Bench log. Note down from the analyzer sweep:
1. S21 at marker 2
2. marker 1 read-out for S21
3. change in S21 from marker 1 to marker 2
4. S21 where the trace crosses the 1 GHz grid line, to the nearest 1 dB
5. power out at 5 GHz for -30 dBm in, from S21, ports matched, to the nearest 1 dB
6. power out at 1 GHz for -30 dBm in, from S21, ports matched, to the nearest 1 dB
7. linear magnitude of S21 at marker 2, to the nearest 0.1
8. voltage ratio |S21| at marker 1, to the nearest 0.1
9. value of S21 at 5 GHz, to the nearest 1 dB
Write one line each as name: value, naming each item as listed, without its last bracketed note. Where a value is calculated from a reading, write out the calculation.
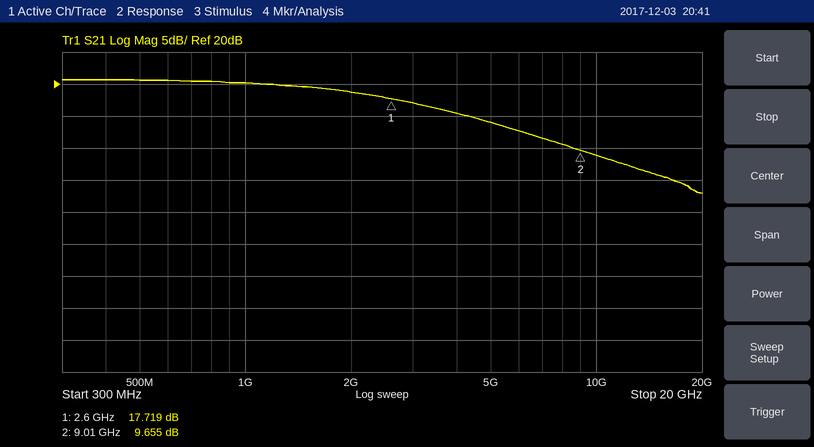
S21 at marker 2: 9.655 dB
marker 1 read-out for S21: 17.719 dB
change in S21 from marker 1 to marker 2: 9.655 − (17.719) = -8.064 dB
S21 where the trace crosses the 1 GHz grid line, to the nearest 1 dB: 20 dB
power out at 5 GHz for -30 dBm in, from S21, ports matched, to the nearest 1 dB: -30 dBm + (14 dB) = -16 dBm
power out at 1 GHz for -30 dBm in, from S21, ports matched, to the nearest 1 dB: -30 dBm + (20 dB) = -10 dBm
linear magnitude of S21 at marker 2, to the nearest 0.1: 10^(9.655/20) ≈ 3.0
voltage ratio |S21| at marker 1, to the nearest 0.1: 10^(17.719/20) ≈ 7.7
value of S21 at 5 GHz, to the nearest 1 dB: 14 dB
